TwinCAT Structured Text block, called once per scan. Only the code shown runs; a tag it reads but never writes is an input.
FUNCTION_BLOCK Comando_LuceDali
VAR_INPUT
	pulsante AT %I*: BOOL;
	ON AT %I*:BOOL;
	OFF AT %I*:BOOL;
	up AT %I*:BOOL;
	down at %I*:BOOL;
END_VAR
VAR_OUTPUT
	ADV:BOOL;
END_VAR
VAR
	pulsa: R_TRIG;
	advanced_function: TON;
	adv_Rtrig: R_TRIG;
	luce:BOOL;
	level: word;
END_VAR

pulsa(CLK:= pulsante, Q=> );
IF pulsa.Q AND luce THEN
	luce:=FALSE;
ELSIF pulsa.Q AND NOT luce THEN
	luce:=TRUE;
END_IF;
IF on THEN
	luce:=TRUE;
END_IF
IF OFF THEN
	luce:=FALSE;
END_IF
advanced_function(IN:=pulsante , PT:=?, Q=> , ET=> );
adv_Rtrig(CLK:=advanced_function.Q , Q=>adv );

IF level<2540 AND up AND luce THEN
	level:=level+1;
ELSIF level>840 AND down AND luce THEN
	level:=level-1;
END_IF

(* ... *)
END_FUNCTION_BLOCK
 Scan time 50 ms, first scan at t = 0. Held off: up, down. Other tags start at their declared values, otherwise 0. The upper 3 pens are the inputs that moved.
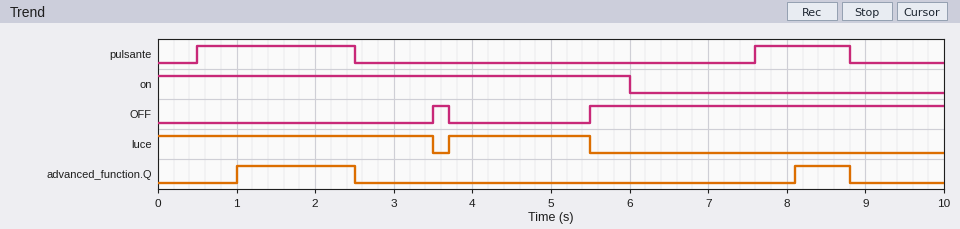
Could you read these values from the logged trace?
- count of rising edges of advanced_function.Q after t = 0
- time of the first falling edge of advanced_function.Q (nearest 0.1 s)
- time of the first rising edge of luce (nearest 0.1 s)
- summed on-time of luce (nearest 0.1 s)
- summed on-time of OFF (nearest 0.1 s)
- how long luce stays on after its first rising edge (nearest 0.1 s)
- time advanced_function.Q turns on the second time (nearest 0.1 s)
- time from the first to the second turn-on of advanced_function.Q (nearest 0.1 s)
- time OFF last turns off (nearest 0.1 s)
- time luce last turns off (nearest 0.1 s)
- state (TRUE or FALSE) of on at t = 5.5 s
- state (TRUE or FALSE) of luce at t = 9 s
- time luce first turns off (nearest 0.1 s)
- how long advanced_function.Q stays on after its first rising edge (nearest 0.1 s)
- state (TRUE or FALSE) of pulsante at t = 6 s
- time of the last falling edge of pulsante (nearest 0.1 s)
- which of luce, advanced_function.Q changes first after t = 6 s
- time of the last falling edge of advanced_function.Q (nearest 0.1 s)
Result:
2
2.5 s
3.7 s
5.3 s
4.7 s
1.8 s
8.1 s
7.1 s
3.7 s
5.5 s
TRUE
FALSE
3.5 s
1.5 s
FALSE
8.8 s
advanced_function.Q
8.8 s
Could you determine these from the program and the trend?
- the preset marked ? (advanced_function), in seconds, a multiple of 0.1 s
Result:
0.5 s
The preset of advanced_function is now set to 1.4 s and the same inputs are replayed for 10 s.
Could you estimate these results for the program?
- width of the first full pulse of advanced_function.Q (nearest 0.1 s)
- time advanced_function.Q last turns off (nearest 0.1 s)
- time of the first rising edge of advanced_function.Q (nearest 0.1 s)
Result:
0.6 s
2.5 s
1.9 s
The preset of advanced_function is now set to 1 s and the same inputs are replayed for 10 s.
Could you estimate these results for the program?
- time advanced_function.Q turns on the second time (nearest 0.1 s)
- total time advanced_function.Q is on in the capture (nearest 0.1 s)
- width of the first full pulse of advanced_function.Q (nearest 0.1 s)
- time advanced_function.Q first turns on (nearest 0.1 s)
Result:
8.6 s
1.2 s
1.0 s
1.5 s
